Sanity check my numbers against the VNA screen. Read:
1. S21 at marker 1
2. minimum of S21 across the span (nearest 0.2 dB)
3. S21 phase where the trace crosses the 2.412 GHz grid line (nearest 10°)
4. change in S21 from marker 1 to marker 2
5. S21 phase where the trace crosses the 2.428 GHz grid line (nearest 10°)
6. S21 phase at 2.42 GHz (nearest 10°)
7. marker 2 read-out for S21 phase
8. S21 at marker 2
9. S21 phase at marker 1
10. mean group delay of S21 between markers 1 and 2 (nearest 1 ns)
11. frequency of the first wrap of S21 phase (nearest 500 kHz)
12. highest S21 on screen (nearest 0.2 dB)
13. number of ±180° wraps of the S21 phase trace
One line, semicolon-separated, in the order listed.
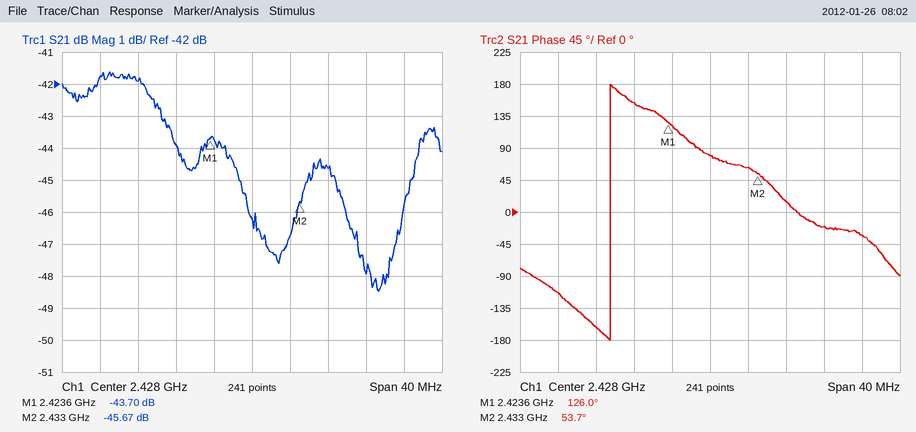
-43.70 dB; -48.4 dB; -110°; -1.97 dB; 80°; 150°; 53.7°; -45.67 dB; 126.0°; 21 ns; 2.4175 GHz; -41.6 dB; 1
